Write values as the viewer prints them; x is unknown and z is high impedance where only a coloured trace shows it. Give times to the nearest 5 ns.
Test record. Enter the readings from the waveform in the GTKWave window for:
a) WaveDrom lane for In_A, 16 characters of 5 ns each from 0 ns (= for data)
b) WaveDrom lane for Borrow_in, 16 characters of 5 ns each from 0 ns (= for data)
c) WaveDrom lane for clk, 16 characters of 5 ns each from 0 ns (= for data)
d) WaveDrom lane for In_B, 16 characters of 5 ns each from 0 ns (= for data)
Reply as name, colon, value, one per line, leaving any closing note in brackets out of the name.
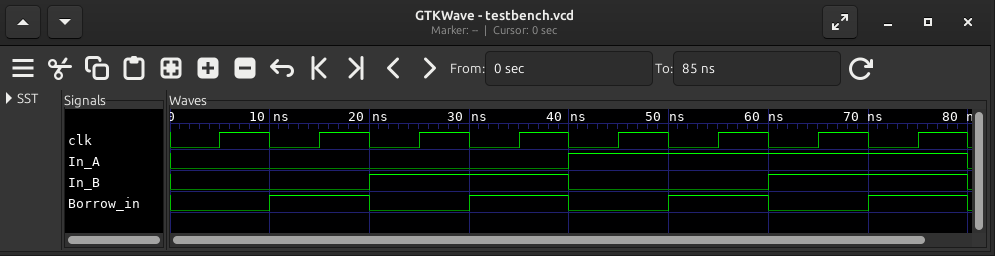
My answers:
WaveDrom lane for In_A, 16 characters of 5 ns each from 0 ns: {name: 'In_A', wave: '0.......1.......'}
WaveDrom lane for Borrow_in, 16 characters of 5 ns each from 0 ns: {name: 'Borrow_in', wave: '0.1.0.1.0.1.0.1.'}
WaveDrom lane for clk, 16 characters of 5 ns each from 0 ns: {name: 'clk', wave: '0101010101010101'}
WaveDrom lane for In_B, 16 characters of 5 ns each from 0 ns: {name: 'In_B', wave: '0...1...0...1...'}
